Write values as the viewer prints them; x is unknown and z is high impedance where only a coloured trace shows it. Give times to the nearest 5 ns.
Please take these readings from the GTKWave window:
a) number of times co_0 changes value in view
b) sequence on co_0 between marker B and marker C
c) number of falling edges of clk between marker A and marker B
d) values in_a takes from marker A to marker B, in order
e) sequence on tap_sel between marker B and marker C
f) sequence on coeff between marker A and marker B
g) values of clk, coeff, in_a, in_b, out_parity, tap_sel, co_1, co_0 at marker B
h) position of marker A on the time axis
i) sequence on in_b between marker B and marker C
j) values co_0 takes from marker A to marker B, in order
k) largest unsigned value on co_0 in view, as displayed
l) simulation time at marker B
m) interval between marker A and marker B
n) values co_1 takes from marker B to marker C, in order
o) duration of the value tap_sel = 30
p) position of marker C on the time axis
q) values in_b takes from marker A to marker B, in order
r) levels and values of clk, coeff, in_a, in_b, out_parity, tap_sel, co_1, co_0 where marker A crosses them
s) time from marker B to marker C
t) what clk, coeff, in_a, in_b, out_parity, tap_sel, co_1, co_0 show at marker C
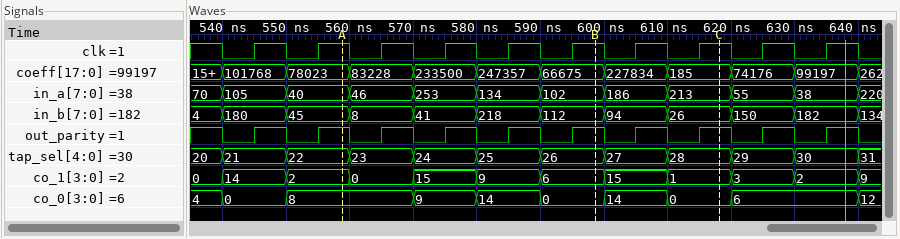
9
0, 14, 0
4
40, 46, 253, 134, 102
26, 27, 28
78023, 83228, 233500, 247357, 66675
clk=1, coeff=66675, in_a=102, in_b=112, out_parity=1, tap_sel=26, co_1=6, co_0=0
560 ns
112, 94, 26
8, 9, 14, 0
14
600 ns
40 ns
6, 15, 1
10 ns
620 ns
45, 8, 41, 218, 112
clk=1, coeff=78023, in_a=40, in_b=45, out_parity=1, tap_sel=22, co_1=2, co_0=8
20 ns
clk=1, coeff=185, in_a=213, in_b=26, out_parity=1, tap_sel=28, co_1=1, co_0=0
